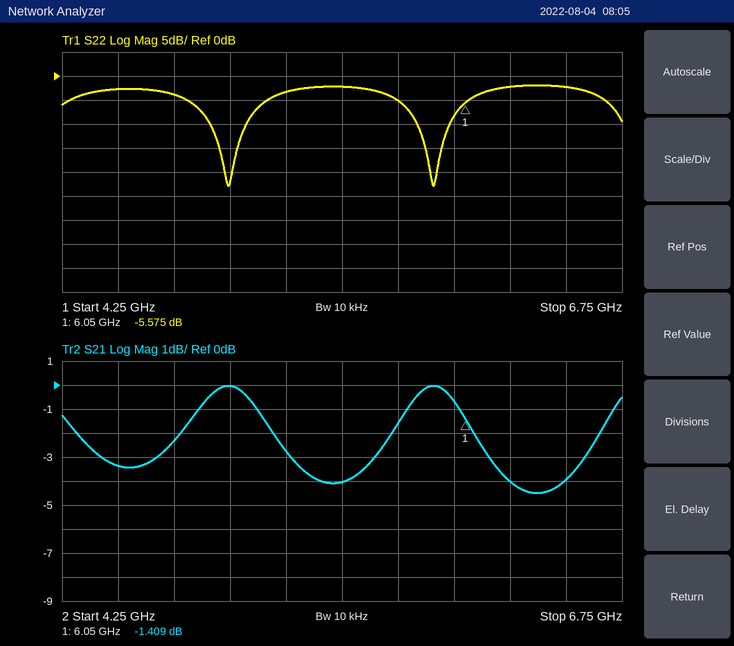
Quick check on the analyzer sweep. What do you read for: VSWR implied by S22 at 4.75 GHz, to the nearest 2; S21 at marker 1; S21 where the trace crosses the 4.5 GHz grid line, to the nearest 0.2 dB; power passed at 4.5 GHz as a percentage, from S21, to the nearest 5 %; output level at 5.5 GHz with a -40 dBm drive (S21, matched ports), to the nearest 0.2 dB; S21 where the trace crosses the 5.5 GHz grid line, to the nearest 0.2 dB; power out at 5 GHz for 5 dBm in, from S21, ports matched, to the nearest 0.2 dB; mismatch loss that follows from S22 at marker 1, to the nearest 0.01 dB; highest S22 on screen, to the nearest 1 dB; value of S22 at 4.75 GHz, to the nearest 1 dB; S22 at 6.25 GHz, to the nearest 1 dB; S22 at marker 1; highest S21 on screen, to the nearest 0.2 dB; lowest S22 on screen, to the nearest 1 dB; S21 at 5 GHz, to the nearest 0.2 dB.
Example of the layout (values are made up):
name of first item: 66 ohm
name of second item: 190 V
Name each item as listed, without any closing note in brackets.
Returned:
VSWR implied by S22 at 4.75 GHz, to the nearest 2: 4
S21 at marker 1: -1.409 dB
S21 where the trace crosses the 4.5 GHz grid line, to the nearest 0.2 dB: -3.4 dB
power passed at 4.5 GHz as a percentage, from S21, to the nearest 5 %: 45 %
output level at 5.5 GHz with a -40 dBm drive (S21, matched ports), to the nearest 0.2 dB: -44.0 dBm
S21 where the trace crosses the 5.5 GHz grid line, to the nearest 0.2 dB: -4.0 dB
power out at 5 GHz for 5 dBm in, from S21, ports matched, to the nearest 0.2 dB: 5.0 dBm
mismatch loss that follows from S22 at marker 1, to the nearest 0.01 dB: 1.41 dB
highest S22 on screen, to the nearest 1 dB: -2 dB
value of S22 at 4.75 GHz, to the nearest 1 dB: -4 dB
S22 at 6.25 GHz, to the nearest 1 dB: -2 dB
S22 at marker 1: -5.575 dB
highest S21 on screen, to the nearest 0.2 dB: 0.0 dB
lowest S22 on screen, to the nearest 1 dB: -23 dB
S21 at 5 GHz, to the nearest 0.2 dB: 0.0 dB
